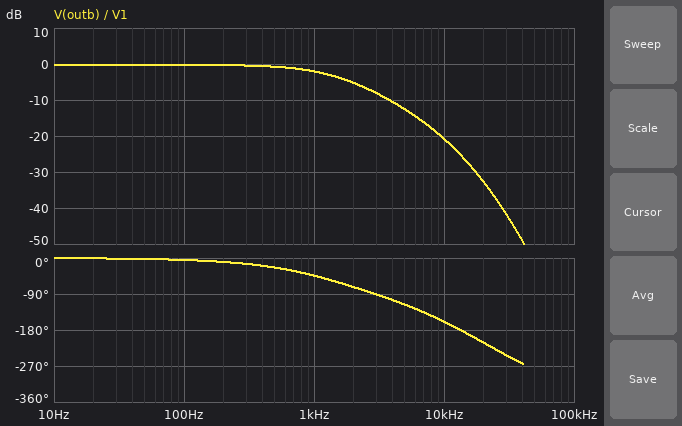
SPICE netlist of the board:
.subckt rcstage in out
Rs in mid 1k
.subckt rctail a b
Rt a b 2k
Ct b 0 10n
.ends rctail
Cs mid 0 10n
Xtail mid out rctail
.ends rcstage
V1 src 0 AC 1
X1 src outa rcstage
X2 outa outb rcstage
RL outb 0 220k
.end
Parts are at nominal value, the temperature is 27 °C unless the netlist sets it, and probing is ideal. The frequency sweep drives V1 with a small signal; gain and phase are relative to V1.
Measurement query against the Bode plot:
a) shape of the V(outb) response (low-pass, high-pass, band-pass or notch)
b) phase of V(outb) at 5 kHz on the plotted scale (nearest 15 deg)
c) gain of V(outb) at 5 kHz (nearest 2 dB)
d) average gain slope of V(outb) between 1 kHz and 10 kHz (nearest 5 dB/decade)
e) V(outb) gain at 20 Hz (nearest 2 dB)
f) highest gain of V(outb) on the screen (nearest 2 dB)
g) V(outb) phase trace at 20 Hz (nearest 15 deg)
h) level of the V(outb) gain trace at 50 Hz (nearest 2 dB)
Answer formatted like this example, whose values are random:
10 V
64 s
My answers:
low-pass
-120 deg
-12 dB
-20 dB/decade
0 dB
0 dB
0 deg
0 dB
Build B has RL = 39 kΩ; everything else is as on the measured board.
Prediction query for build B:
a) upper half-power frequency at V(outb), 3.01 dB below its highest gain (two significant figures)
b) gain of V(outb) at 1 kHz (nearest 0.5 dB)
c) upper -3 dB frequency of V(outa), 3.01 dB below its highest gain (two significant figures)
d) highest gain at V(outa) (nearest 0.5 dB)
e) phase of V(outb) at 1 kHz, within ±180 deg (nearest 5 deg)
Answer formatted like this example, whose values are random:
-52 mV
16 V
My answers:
1.5 kHz
-3.0 dB
1.7 kHz
-0.5 dB
-40 deg
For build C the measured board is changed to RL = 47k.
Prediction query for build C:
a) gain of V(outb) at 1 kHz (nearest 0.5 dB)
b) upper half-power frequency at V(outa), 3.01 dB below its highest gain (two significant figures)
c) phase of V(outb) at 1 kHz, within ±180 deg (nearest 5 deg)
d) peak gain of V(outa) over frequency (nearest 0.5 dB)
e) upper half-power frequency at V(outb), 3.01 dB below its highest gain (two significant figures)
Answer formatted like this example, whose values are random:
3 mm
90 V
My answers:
-2.5 dB
1.7 kHz
-40 deg
-0.5 dB
1.5 kHz
